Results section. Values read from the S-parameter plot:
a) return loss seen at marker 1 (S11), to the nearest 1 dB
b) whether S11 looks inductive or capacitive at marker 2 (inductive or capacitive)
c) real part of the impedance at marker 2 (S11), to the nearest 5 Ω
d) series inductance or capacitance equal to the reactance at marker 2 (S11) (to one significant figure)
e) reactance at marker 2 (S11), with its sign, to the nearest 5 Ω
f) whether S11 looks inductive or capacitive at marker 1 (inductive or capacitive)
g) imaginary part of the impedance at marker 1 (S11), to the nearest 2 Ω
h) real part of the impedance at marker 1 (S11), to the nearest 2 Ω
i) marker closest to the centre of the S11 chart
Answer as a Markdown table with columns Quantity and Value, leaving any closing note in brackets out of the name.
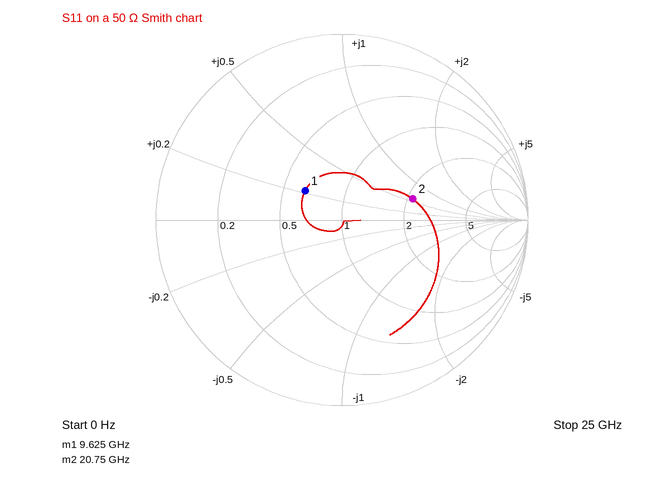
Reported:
| Quantity | Value |
|---|---|
| return loss seen at marker 1 (S11), to the nearest 1 dB | 12 dB |
| whether S11 looks inductive or capacitive at marker 2 | inductive |
| real part of the impedance at marker 2 (S11), to the nearest 5 Ω | 105 Ω |
| series inductance or capacitance equal to the reactance at marker 2 (S11) | 200 pH |
| reactance at marker 2 (S11), with its sign, to the nearest 5 Ω | +30 Ω |
| whether S11 looks inductive or capacitive at marker 1 | inductive |
| imaginary part of the impedance at marker 1 (S11), to the nearest 2 Ω | +10 Ω |
| real part of the impedance at marker 1 (S11), to the nearest 2 Ω | 32 Ω |
| marker closest to the centre of the S11 chart | marker 1 |
